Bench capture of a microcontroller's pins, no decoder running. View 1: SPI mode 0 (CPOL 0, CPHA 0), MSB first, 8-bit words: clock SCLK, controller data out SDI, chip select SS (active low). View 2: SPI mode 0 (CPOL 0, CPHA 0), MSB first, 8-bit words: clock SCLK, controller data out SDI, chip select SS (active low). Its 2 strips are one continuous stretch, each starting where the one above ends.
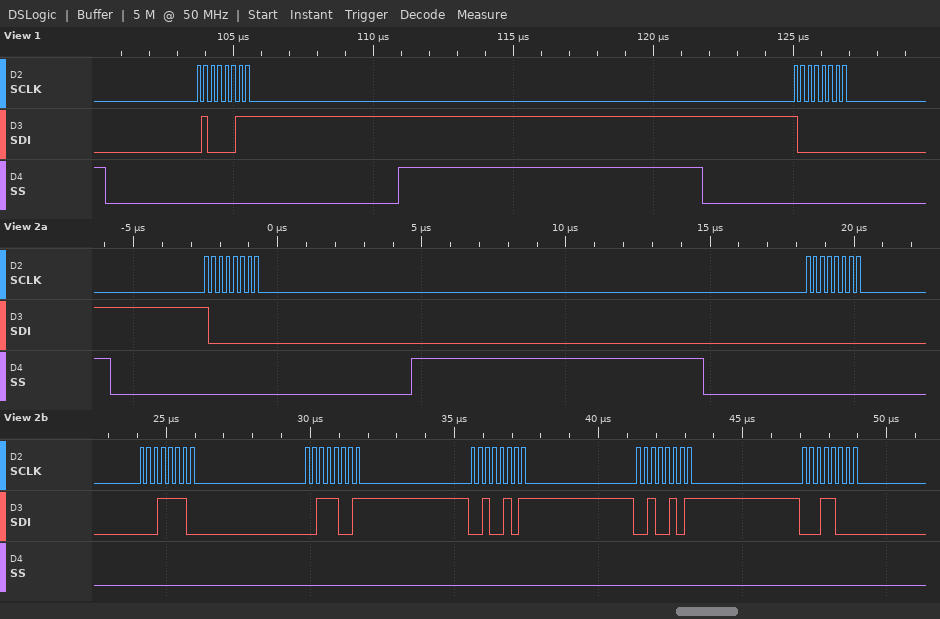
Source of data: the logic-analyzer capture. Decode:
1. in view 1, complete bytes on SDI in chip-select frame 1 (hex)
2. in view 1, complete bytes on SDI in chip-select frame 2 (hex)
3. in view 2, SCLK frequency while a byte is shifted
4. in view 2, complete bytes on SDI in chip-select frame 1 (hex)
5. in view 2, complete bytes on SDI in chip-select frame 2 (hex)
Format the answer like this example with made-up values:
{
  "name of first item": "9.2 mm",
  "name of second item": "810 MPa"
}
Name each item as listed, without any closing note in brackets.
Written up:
{
  "in view 1, complete bytes on SDI in chip-select frame 1": "43",
  "in view 1, complete bytes on SDI in chip-select frame 2": "80",
  "in view 2, SCLK frequency while a byte is shifted": "4 MHz",
  "in view 2, complete bytes on SDI in chip-select frame 1": "80",
  "in view 2, complete bytes on SDI in chip-select frame 2": "00 1E 39 25 25 18"
}
